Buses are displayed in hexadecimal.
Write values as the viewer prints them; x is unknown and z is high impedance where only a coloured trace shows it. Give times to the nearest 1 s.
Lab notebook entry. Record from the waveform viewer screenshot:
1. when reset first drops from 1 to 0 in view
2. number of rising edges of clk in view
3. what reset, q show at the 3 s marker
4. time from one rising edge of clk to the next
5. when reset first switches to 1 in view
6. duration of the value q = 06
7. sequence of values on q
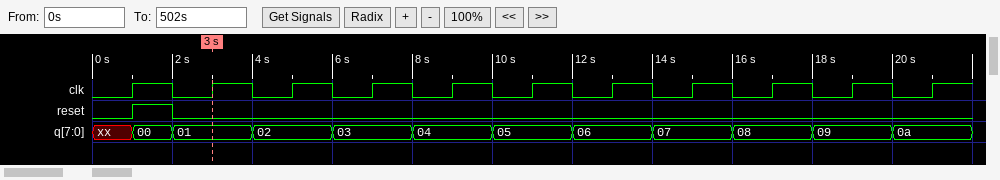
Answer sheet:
2 s
11
reset=0, q=01
2 s
1 s
2 s
xx, 00, 01, 02, 03, 04, 05, 06, 07, 08, 09, 0a
